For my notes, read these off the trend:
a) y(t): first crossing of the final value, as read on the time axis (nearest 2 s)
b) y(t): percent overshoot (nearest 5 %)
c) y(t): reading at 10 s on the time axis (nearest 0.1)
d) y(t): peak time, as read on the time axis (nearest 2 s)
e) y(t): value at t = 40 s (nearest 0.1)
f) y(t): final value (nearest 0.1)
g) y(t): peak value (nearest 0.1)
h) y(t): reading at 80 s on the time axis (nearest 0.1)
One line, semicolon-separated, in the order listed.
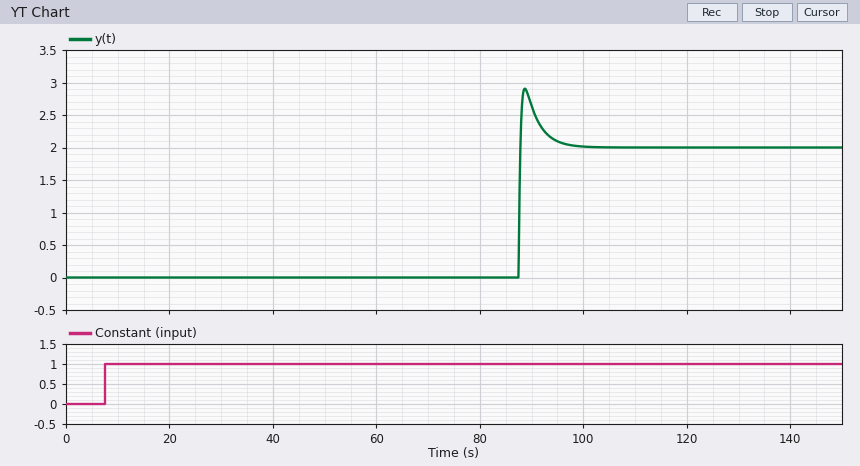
88 s; 45 %; 0.0; 88 s; 0.0; 2.0; 2.9; 0.0
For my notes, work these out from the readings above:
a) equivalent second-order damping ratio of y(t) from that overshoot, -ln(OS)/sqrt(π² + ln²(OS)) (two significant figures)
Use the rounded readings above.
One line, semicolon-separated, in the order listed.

0.25
